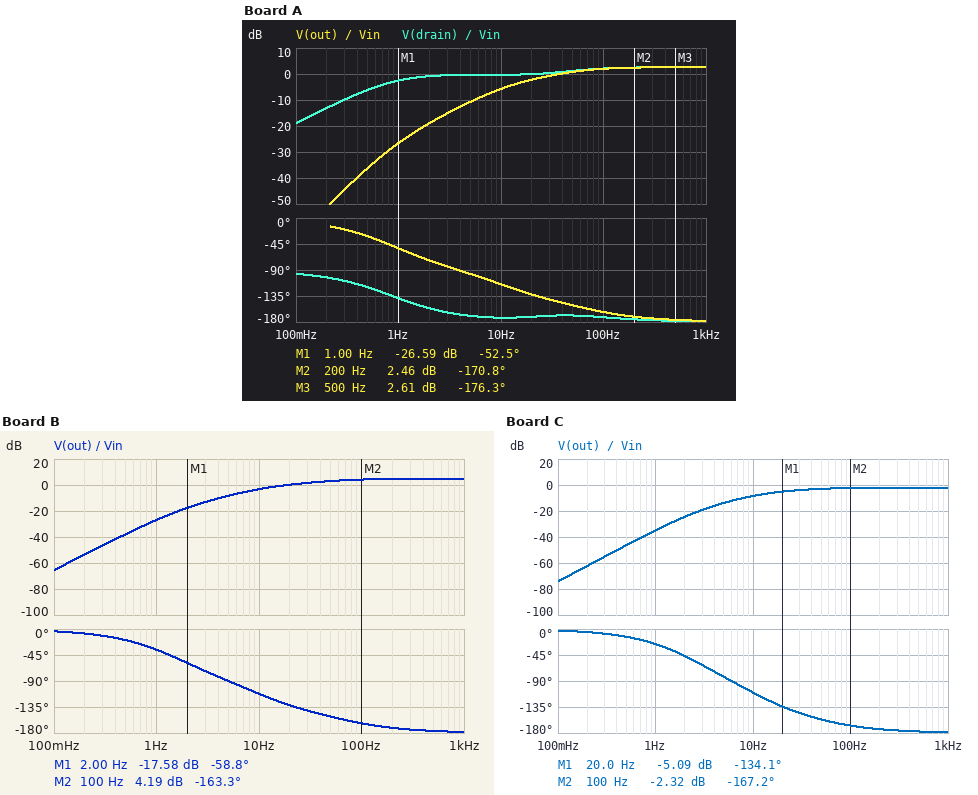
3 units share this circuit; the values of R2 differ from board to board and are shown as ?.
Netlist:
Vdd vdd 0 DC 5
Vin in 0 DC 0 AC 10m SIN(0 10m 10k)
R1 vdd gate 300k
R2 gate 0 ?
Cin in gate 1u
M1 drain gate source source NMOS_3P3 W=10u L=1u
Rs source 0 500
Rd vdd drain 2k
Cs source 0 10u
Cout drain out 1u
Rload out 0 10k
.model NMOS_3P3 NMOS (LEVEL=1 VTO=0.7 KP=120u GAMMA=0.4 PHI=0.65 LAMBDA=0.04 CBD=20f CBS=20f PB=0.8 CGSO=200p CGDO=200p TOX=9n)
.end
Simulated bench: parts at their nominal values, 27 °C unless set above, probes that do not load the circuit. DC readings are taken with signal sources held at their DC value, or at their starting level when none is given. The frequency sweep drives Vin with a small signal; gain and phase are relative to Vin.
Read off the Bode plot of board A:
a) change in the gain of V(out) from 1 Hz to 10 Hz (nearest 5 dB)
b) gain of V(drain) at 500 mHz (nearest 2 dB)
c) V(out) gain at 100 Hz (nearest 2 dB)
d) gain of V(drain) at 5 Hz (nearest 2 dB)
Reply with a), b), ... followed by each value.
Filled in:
a) 20 dB
b) -6 dB
c) 2 dB
d) 0 dB
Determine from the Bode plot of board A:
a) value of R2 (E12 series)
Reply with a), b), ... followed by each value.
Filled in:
a) 470 kΩ
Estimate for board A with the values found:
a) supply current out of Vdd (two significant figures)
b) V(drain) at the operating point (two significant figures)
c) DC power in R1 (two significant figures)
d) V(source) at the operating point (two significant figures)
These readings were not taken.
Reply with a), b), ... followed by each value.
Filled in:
a) 1.5 mA
b) 2.0 V
c) 13 µW
d) 760 mV
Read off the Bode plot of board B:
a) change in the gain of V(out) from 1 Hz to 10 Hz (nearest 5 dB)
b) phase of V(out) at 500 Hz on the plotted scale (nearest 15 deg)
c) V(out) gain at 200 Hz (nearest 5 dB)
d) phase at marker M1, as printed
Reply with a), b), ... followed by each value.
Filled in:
a) 25 dB
b) -180 deg
c) 5 dB
d) -58.8 deg
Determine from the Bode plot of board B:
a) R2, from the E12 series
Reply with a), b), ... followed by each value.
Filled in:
a) 150 kΩ
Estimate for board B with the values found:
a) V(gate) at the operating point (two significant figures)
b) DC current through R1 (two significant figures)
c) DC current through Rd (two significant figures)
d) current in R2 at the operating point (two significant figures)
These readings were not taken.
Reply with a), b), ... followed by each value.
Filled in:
a) 1.7 V
b) 11 µA
c) 410 µA
d) 11 µA
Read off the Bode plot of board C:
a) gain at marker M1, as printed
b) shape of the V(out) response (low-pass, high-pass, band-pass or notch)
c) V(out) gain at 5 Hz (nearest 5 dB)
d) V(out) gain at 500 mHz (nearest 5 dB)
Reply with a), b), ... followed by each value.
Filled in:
a) -5.09 dB
b) high-pass
c) -15 dB
d) -45 dB
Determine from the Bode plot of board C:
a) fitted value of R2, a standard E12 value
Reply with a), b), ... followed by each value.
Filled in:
a) 82 kΩ
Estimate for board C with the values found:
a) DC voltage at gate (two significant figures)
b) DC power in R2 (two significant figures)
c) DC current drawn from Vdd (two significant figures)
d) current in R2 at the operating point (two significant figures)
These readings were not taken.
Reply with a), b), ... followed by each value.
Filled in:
a) 1.1 V
b) 14 µW
c) 93 µA
d) 13 µA
